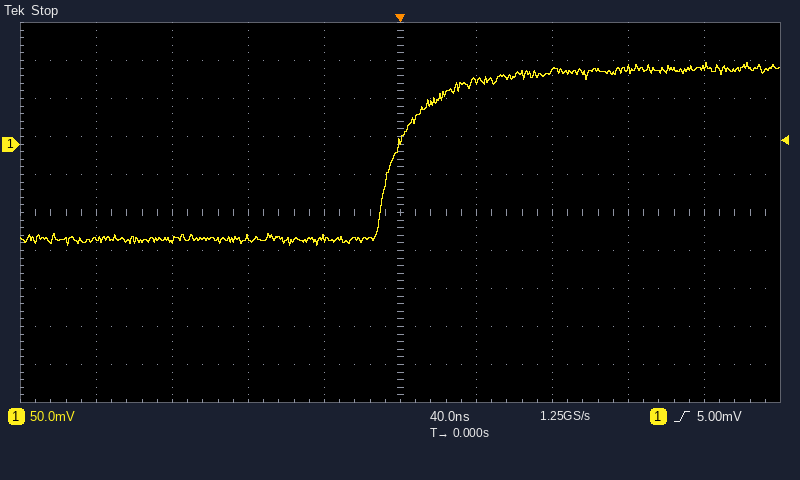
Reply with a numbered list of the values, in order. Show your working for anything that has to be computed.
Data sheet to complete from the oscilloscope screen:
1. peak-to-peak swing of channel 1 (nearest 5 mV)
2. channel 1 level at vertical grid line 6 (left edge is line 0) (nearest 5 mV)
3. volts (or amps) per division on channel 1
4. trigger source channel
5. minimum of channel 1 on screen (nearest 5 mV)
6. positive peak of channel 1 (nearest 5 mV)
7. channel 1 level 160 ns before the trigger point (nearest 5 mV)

1. 105 mV − (-135 mV) = 240 mV
2. 85 mV
3. 50 mV
4. channel 1
5. -135 mV
6. 105 mV
7. -125 mV
